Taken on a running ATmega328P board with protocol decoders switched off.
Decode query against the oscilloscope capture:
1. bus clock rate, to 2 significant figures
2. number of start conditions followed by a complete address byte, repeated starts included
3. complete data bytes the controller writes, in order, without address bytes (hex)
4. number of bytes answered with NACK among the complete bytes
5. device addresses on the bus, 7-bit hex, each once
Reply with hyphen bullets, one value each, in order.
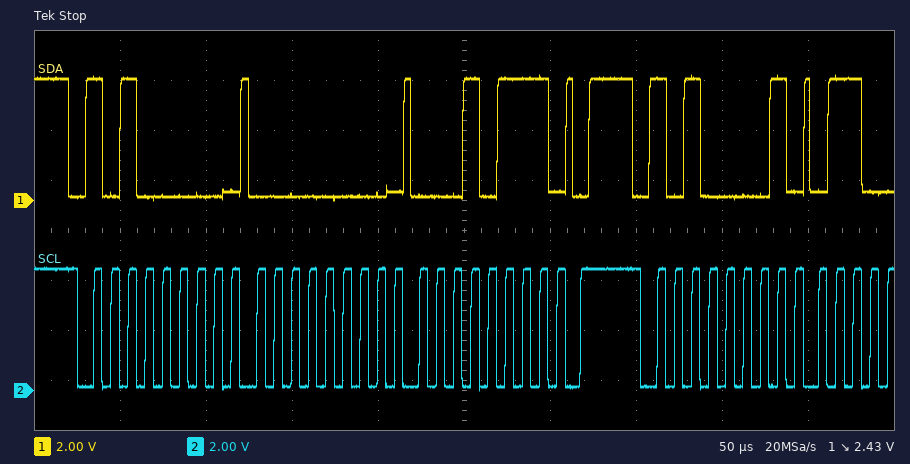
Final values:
- 100 kHz
- 2
- 00 17
- 0
- 0x50
